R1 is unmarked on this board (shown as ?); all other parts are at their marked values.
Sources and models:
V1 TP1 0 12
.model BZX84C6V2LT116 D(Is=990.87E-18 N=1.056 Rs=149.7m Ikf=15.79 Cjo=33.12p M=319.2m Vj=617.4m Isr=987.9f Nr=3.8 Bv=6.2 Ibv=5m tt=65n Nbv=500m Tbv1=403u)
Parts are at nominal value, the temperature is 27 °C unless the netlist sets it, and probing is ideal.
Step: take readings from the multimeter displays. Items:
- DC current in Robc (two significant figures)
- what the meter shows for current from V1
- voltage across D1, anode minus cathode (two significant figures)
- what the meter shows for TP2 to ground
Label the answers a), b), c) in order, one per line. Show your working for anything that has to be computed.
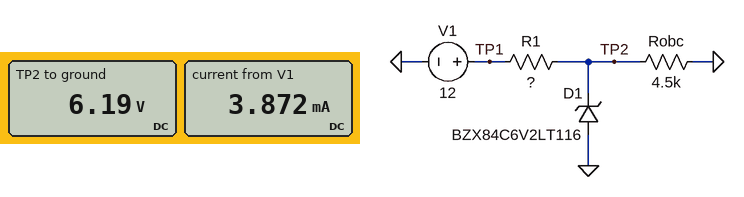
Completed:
a) (6.19 V) / 4.5 kΩ = 1.4 mA
b) 3.872 mA
c) 0 V - 6.19 V = -6.2 V
d) 6.19 V
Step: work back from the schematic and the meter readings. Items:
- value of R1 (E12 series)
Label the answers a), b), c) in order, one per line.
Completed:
a) 1.5 kΩ
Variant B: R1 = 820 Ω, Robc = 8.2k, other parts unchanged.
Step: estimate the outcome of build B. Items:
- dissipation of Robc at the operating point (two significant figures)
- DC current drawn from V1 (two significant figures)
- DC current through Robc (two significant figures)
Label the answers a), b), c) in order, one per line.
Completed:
a) 4.7 mW
b) 7.1 mA
c) 760 µA
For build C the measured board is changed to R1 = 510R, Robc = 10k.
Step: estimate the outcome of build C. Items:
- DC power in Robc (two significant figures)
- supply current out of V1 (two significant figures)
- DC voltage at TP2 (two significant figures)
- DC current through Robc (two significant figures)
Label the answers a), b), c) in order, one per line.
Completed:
a) 3.9 mW
b) 11 mA
c) 6.2 V
d) 620 µA
